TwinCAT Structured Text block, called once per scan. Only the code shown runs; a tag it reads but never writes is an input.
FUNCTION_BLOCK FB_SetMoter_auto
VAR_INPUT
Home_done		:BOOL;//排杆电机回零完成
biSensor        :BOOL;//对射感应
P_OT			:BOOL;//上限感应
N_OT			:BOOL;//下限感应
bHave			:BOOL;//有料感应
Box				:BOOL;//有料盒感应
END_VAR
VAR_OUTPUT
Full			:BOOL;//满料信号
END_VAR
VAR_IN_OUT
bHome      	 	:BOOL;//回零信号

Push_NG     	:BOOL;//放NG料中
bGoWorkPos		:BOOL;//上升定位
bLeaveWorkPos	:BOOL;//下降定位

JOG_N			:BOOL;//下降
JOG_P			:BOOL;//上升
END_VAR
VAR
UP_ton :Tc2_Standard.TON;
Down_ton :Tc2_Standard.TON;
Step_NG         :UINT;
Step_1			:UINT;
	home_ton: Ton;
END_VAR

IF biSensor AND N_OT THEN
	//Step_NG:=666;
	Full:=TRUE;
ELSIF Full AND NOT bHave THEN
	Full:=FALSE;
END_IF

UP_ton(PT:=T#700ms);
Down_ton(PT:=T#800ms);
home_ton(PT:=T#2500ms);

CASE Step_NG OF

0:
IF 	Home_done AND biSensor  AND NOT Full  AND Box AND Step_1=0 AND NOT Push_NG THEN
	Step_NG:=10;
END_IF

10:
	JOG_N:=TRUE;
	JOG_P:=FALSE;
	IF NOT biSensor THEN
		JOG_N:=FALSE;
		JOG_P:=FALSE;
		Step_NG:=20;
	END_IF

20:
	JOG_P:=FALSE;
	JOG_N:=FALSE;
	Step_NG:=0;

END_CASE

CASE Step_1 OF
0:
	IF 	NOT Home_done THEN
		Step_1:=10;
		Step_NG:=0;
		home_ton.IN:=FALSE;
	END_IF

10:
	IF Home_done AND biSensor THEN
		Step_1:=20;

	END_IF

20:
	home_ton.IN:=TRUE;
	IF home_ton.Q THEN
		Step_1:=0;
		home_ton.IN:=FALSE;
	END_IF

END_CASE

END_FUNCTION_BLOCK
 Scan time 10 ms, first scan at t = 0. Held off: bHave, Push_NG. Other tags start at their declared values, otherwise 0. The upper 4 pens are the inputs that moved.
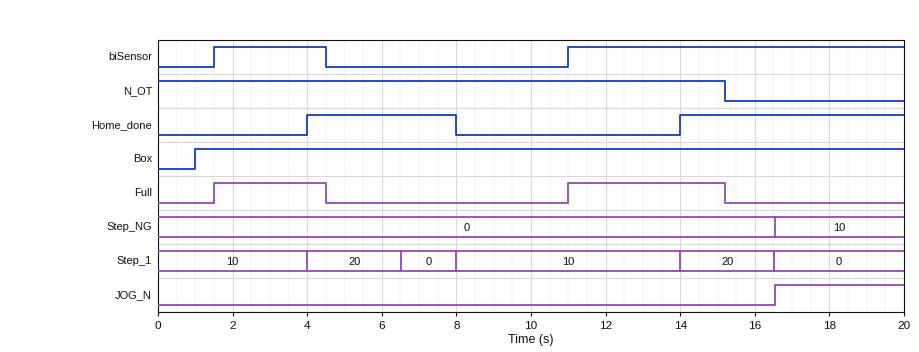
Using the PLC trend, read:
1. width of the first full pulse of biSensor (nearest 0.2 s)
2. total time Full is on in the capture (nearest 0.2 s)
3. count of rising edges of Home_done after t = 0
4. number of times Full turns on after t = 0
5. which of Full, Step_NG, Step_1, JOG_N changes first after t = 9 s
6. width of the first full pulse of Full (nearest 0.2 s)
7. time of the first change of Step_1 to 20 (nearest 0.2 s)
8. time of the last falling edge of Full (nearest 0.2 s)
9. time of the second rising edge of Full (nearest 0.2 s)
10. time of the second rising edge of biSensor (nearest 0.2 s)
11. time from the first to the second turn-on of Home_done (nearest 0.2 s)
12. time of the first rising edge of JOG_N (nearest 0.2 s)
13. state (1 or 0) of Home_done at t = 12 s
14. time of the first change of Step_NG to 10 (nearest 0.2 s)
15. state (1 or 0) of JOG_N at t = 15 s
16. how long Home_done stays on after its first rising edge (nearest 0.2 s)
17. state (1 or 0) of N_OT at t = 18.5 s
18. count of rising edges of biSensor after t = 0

3.0 s
7.2 s
2
2
Full
3.0 s
4.0 s
15.2 s
11.0 s
11.0 s
10.0 s
16.6 s
0
16.6 s
0
4.0 s
0
2
